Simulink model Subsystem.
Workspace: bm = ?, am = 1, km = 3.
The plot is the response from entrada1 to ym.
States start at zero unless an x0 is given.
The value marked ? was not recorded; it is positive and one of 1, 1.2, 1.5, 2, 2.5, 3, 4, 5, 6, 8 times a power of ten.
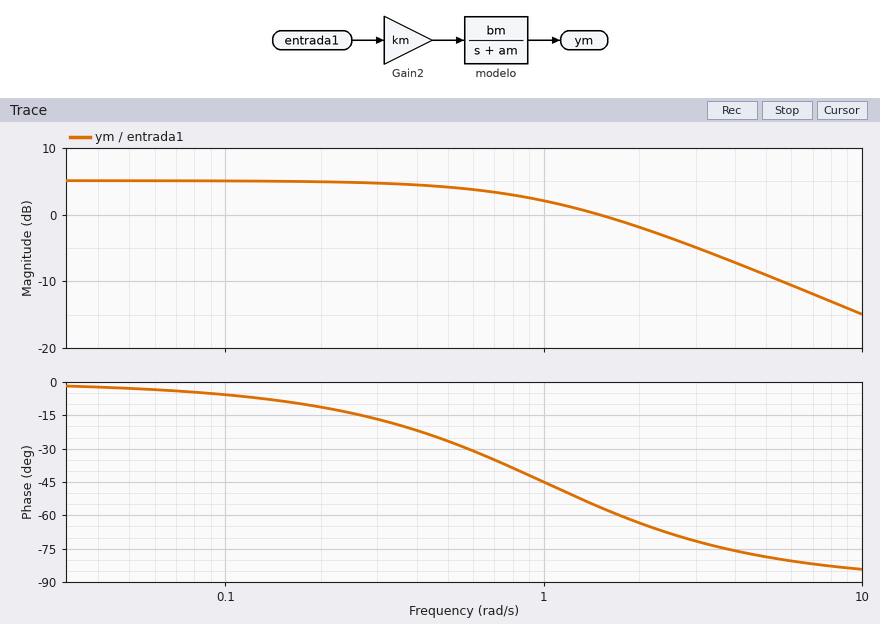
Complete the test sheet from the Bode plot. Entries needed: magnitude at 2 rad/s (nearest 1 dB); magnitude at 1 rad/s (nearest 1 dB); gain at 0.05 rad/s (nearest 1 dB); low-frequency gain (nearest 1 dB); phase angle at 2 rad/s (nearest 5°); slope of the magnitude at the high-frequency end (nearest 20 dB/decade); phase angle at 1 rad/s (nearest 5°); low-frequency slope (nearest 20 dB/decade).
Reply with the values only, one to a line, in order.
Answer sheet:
-2 dB
2 dB
5 dB
5 dB
-65°
-20 dB/decade
-45°
0 dB/decade
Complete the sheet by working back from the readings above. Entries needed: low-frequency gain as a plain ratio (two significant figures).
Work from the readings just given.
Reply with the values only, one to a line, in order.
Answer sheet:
1.8
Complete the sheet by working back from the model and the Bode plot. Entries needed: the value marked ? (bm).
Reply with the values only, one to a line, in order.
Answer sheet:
0.6
